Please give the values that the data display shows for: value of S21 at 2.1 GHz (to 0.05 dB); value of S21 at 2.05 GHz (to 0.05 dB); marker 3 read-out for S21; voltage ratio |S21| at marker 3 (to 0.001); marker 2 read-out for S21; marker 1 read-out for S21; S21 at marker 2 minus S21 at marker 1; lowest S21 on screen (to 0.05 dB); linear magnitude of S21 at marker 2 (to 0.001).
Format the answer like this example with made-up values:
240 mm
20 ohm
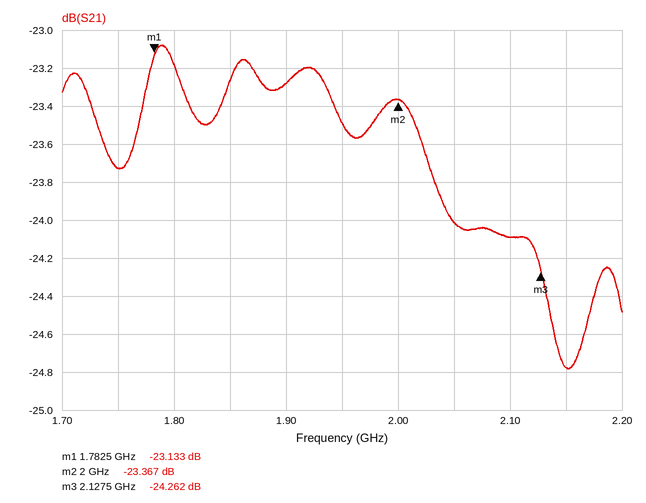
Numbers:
-24.10 dB
-24.00 dB
-24.262 dB
0.061
-23.367 dB
-23.133 dB
-0.234 dB
-24.80 dB
0.068
